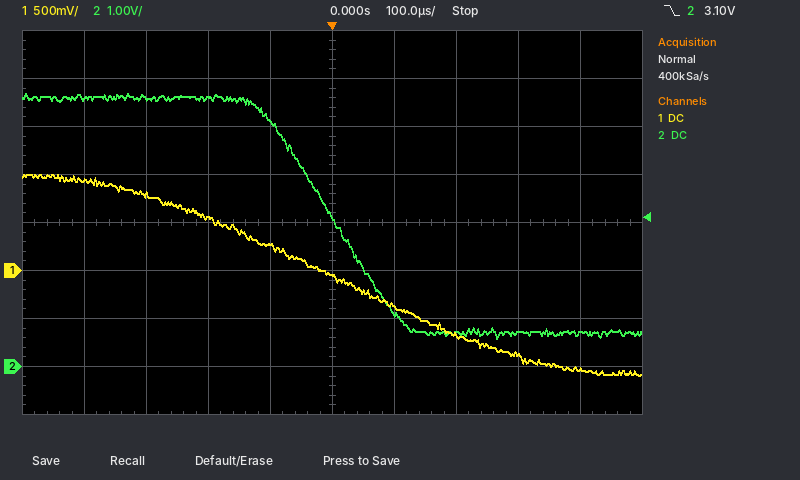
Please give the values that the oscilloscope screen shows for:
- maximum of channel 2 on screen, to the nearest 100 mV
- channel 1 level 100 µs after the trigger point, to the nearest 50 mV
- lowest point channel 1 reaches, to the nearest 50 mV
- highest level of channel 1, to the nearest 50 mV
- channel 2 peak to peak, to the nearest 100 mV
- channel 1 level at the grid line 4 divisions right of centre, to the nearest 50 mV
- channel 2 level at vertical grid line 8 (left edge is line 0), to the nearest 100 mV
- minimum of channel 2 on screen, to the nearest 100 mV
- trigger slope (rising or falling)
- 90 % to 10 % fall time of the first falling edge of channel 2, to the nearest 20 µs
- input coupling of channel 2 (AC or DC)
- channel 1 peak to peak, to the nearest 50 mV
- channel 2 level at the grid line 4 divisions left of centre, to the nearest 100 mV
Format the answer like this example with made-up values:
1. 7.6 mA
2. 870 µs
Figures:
1. 5.7 V
2. -350 mV
3. -1.10 V
4. 1.00 V
5. 5.1 V
6. -1.05 V
7. 700 mV
8. 600 mV
9. falling
10. 200 µs
11. DC
12. 2.10 V
13. 5.6 V
